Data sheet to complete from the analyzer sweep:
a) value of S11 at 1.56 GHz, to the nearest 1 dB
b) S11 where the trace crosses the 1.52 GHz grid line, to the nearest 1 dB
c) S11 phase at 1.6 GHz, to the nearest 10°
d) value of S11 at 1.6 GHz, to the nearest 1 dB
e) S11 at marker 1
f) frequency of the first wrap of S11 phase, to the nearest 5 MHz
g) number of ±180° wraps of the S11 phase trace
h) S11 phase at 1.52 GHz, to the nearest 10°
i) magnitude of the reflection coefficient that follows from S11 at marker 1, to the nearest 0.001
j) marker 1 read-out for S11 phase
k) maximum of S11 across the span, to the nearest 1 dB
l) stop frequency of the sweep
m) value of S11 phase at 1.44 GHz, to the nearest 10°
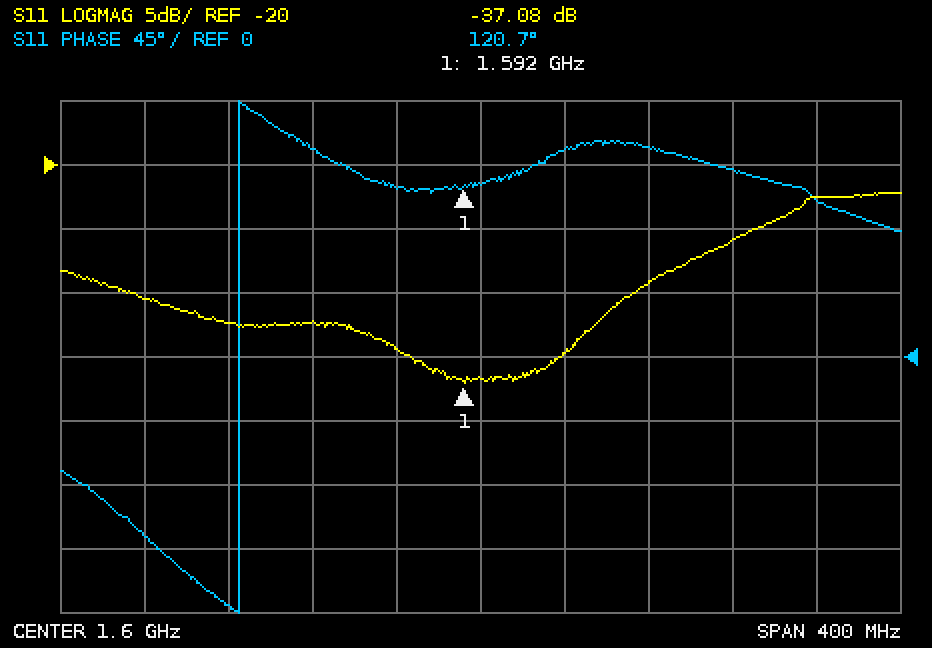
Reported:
-34 dB
-32 dB
120°
-37 dB
-37.08 dB
1.485 GHz
1
150°
0.014
120.7°
-22 dB
1.8 GHz
-130°
